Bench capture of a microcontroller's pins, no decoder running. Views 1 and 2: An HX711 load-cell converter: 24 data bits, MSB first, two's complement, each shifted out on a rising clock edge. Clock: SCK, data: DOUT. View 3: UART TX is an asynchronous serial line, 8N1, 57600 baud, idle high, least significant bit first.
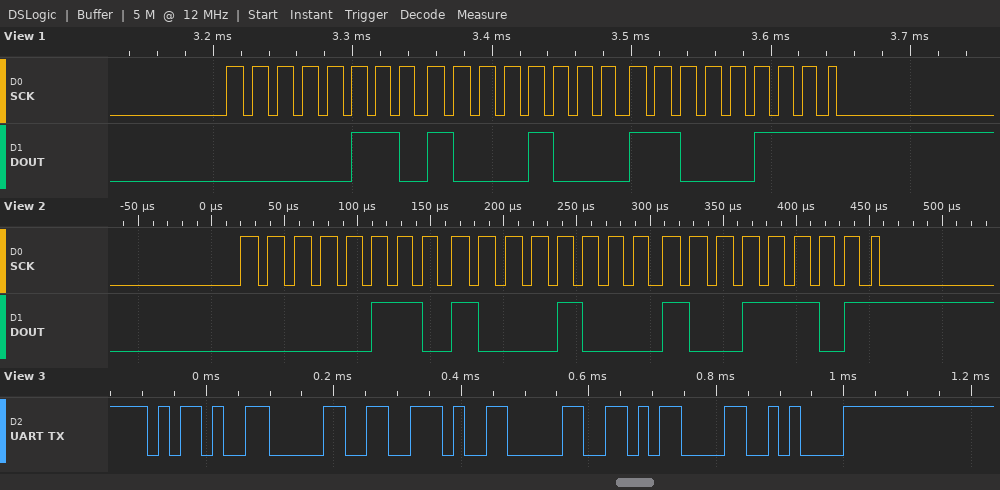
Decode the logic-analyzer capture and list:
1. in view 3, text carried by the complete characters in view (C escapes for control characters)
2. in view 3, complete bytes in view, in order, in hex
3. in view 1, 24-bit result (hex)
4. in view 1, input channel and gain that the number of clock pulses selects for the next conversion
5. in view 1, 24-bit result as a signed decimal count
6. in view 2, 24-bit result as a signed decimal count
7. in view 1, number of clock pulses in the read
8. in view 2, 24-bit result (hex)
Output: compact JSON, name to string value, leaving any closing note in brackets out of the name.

{"in view 3, text carried by the complete characters in view": "\"-0.0\\r\\n\"", "in view 3, complete bytes in view, in order, in hex": "2D 30 2E 30 0D 0A", "in view 1, 24-bit result": "0x0688C7", "in view 1, input channel and gain that the number of clock pulses selects for the next conversion": "channel A, gain 128", "in view 1, 24-bit result as a signed decimal count": "428231", "in view 2, 24-bit result as a signed decimal count": "428189", "in view 1, number of clock pulses in the read": "25", "in view 2, 24-bit result": "0x06889D"}
